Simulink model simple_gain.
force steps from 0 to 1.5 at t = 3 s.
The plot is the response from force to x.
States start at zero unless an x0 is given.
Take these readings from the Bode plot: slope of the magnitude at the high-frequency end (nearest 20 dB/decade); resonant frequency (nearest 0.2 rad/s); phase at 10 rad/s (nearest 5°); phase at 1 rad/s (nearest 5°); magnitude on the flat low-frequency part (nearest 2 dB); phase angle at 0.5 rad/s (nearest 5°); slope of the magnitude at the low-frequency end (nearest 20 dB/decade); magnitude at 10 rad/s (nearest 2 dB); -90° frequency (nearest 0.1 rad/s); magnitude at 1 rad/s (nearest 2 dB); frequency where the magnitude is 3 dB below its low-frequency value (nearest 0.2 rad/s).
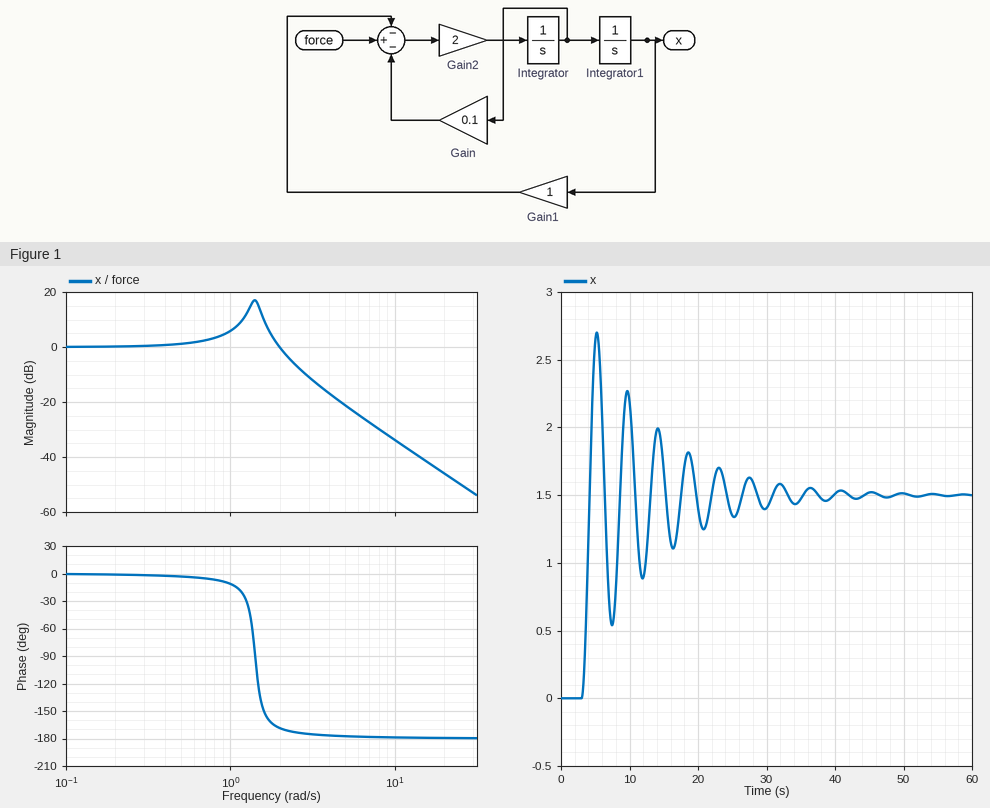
-40 dB/decade
1.4 rad/s
-180°
-10°
0 dB
-5°
0 dB/decade
-34 dB
1.4 rad/s
6 dB
2.2 rad/s
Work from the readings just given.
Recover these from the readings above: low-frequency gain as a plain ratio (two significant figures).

1.0
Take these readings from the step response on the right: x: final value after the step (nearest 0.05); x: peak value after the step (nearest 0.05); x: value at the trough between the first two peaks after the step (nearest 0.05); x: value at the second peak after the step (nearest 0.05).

1.50
2.70
0.55
2.25
